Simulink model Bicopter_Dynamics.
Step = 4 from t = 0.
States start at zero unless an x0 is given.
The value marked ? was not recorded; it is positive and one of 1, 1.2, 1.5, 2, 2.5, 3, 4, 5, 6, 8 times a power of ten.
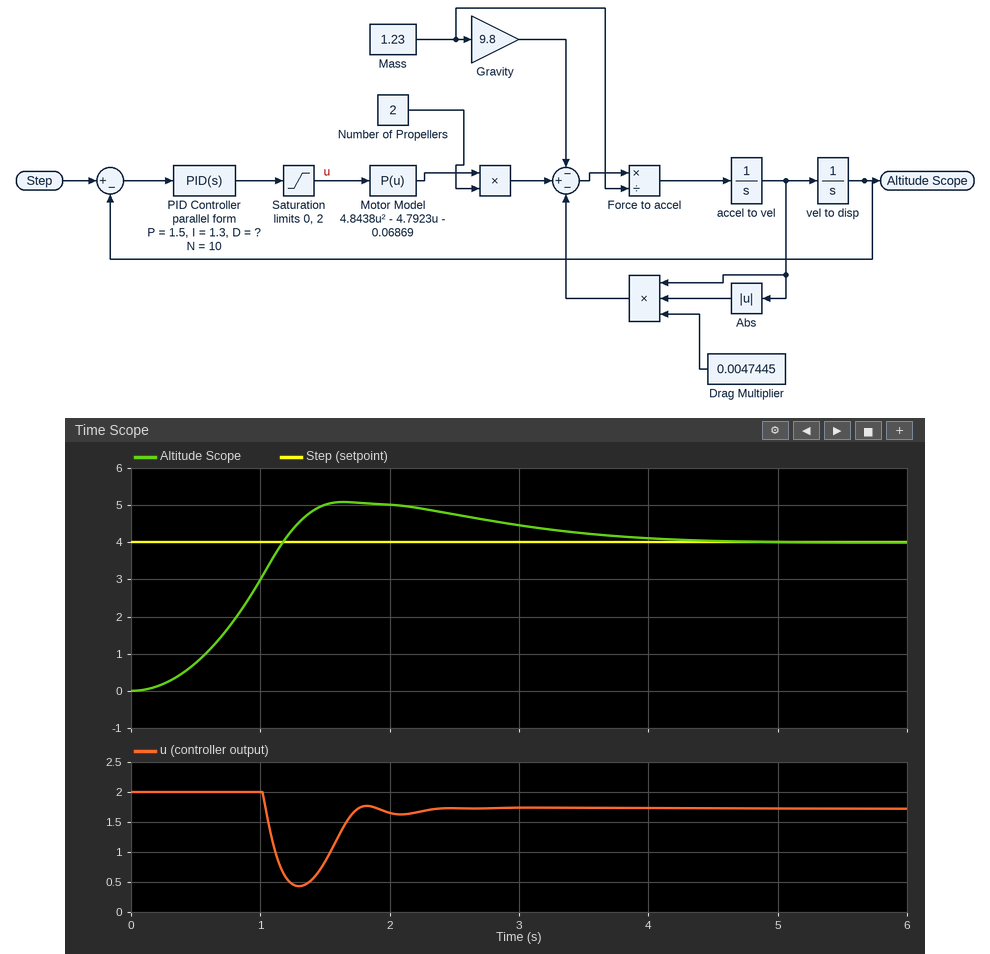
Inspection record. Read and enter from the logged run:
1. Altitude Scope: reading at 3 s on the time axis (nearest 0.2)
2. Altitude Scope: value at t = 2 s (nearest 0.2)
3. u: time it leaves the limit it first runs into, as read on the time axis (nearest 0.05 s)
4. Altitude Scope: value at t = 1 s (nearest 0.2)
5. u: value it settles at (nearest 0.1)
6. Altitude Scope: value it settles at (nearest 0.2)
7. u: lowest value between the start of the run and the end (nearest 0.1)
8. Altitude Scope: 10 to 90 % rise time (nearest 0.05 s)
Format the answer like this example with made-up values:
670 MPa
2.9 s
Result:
4.4
5.0
1.00 s
3.0
1.7
4.0
0.4
0.75 s
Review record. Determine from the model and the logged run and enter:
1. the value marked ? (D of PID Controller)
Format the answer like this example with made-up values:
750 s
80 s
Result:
0.6
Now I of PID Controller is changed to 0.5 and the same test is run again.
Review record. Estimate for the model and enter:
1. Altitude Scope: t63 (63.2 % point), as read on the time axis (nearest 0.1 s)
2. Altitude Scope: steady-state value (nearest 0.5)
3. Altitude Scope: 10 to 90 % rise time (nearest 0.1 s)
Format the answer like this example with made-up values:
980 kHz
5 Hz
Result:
0.9 s
4.0
1.2 s
